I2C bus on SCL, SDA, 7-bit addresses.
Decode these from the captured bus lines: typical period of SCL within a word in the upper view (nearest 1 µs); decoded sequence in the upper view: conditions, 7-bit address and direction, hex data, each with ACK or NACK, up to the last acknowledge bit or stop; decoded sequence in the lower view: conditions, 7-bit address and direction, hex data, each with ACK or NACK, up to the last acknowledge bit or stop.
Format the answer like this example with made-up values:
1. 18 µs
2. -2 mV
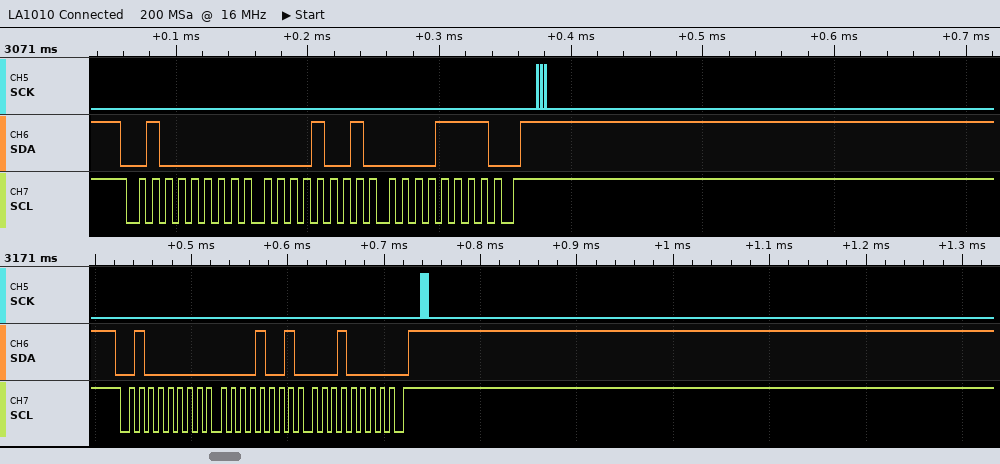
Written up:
1. 10 µs
2. start, address 20 write ACK, 09 ACK, 0F ACK, stop
3. start, address 20 write ACK, 09 ACK, 10 ACK, stop
